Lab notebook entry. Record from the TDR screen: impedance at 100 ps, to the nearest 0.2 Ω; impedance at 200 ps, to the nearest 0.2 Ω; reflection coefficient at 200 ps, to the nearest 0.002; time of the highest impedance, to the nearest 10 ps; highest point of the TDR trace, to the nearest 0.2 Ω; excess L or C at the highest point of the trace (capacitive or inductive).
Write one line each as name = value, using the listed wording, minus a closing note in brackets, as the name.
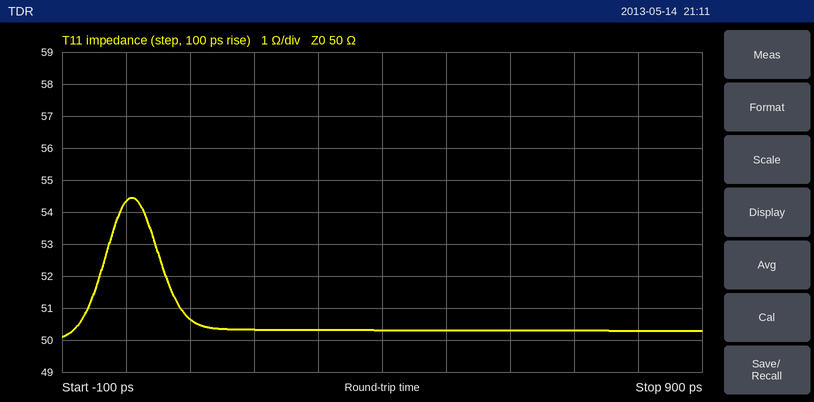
impedance at 100 ps, to the nearest 0.2 Ω = 50.6 Ω
impedance at 200 ps, to the nearest 0.2 Ω = 50.4 Ω
reflection coefficient at 200 ps, to the nearest 0.002 = +0.004
time of the highest impedance, to the nearest 10 ps = 10 ps
highest point of the TDR trace, to the nearest 0.2 Ω = 54.4 Ω
excess L or C at the highest point of the trace = inductive
